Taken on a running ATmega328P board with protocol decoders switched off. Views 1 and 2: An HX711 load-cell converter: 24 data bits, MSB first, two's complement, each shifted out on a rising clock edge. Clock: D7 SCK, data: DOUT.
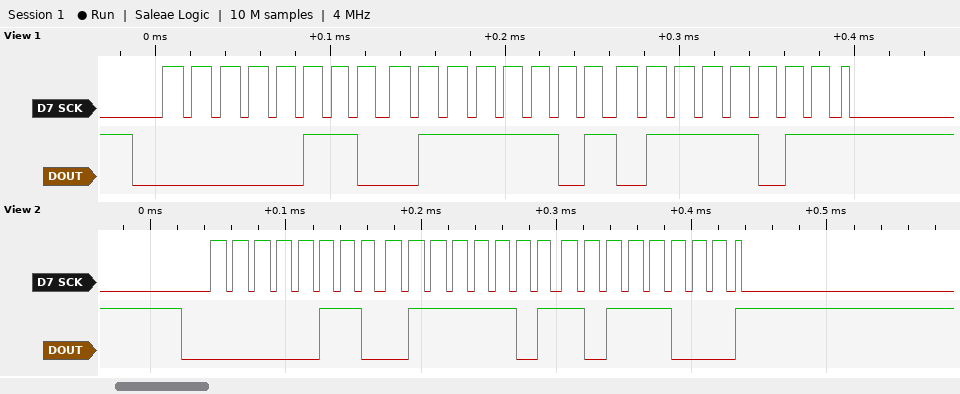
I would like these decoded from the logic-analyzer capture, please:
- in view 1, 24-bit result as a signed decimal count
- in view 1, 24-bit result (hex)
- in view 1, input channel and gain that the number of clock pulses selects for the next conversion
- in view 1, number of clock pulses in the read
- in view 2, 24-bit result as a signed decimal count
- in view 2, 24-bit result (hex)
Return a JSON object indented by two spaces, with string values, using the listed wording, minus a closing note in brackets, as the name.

{
  "in view 1, 24-bit result as a signed decimal count": "425339",
  "in view 1, 24-bit result": "0x067D7B",
  "in view 1, input channel and gain that the number of clock pulses selects for the next conversion": "channel A, gain 128",
  "in view 1, number of clock pulses in the read": "25",
  "in view 2, 24-bit result as a signed decimal count": "425400",
  "in view 2, 24-bit result": "0x067DB8"
}
